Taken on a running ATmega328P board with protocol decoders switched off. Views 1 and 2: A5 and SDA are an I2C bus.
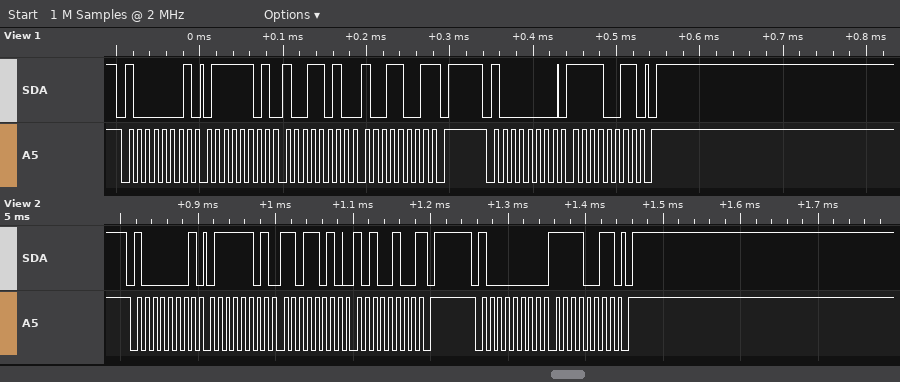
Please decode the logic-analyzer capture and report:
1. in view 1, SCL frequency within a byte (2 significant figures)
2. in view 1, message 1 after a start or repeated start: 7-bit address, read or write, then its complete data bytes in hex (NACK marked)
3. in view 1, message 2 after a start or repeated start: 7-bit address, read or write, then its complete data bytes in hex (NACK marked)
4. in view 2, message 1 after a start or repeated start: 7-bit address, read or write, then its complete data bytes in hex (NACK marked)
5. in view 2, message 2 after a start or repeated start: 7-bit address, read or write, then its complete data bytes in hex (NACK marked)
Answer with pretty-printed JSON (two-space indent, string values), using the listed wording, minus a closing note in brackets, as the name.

{
  "in view 1, SCL frequency within a byte": "100 kHz",
  "in view 1, message 1 after a start or repeated start: 7-bit address, read or write, then its complete data bytes in hex": "0x40 read: 7D 9A 99 NACK",
  "in view 1, message 2 after a start or repeated start: 7-bit address, read or write, then its complete data bytes in hex": "0x40 write: F3",
  "in view 2, message 1 after a start or repeated start: 7-bit address, read or write, then its complete data bytes in hex": "0x40 read: 7D DA A4 NACK",
  "in view 2, message 2 after a start or repeated start: 7-bit address, read or write, then its complete data bytes in hex": "0x40 write: F3"
}
